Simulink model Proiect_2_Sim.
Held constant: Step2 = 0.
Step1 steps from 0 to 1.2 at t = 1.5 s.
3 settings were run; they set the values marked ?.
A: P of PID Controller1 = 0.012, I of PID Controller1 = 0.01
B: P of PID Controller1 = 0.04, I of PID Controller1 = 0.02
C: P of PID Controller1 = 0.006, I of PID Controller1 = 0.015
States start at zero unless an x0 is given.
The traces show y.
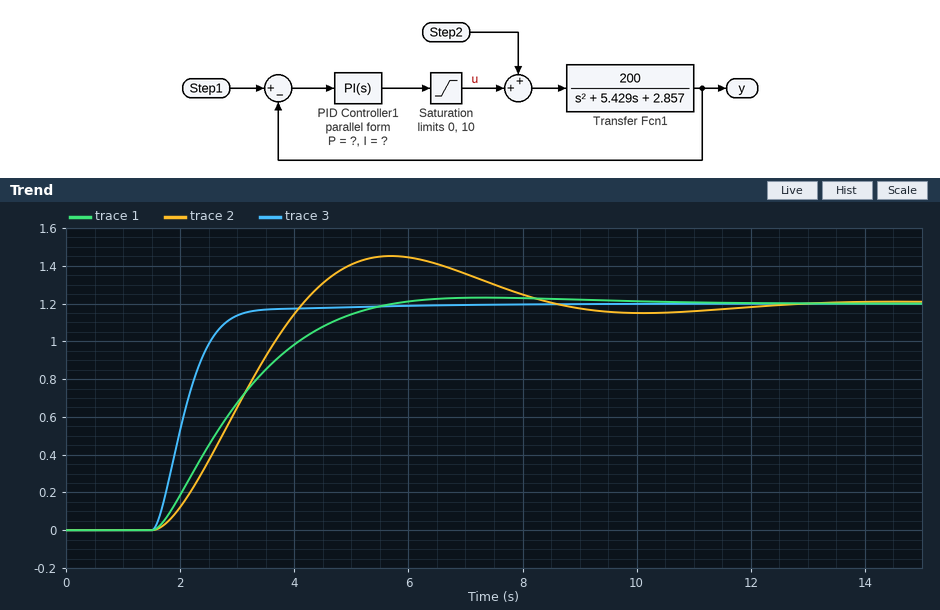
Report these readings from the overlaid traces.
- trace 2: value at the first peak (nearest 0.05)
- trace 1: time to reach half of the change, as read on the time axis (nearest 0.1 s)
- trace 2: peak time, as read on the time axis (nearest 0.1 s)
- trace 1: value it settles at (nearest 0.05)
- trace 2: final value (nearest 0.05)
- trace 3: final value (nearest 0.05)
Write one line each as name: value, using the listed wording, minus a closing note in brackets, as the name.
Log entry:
trace 2: value at the first peak: 1.45
trace 1: time to reach half of the change, as read on the time axis: 2.8 s
trace 2: peak time, as read on the time axis: 5.7 s
trace 1: value it settles at: 1.20
trace 2: final value: 1.20
trace 3: final value: 1.20
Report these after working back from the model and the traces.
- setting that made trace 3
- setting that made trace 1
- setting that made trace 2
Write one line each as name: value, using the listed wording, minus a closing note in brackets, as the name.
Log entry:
setting that made trace 3: B
setting that made trace 1: A
setting that made trace 2: C
